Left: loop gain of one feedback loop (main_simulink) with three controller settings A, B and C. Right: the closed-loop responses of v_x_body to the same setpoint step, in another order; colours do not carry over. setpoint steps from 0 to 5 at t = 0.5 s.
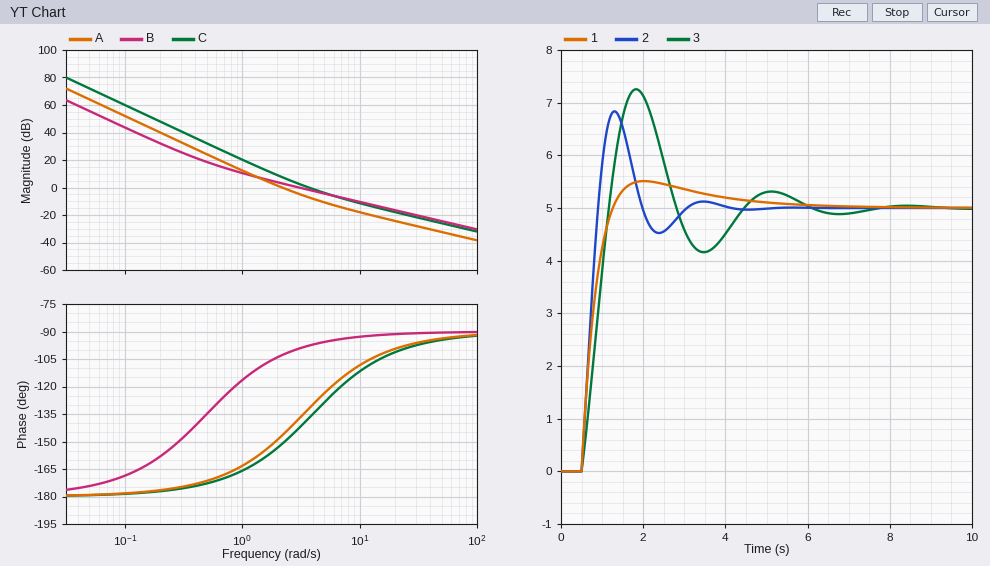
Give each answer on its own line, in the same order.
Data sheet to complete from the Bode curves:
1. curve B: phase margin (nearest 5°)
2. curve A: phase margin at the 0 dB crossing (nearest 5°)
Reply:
80°
35°
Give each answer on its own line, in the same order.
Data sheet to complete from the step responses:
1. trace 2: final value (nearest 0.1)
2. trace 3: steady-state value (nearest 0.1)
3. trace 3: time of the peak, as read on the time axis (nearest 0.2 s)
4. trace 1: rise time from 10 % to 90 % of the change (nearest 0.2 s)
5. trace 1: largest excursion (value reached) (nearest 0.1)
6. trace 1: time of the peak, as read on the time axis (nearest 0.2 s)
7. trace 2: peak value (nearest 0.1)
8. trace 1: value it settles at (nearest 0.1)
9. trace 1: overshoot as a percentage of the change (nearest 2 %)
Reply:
5.0
5.0
1.8 s
0.6 s
5.5
2.0 s
6.8
5.0
10 %
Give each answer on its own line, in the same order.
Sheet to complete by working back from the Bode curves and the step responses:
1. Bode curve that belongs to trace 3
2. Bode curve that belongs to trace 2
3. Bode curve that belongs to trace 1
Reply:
A
C
B
